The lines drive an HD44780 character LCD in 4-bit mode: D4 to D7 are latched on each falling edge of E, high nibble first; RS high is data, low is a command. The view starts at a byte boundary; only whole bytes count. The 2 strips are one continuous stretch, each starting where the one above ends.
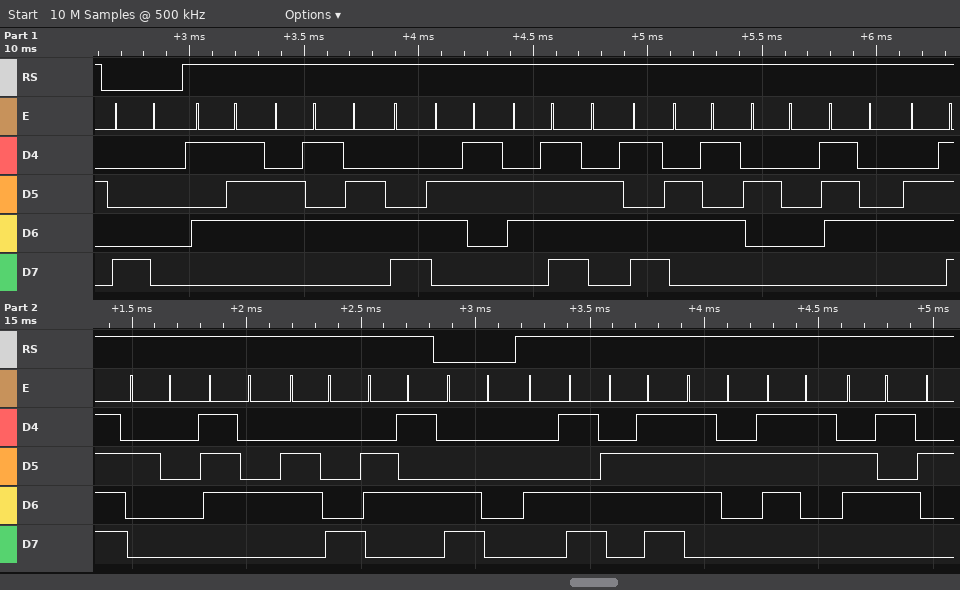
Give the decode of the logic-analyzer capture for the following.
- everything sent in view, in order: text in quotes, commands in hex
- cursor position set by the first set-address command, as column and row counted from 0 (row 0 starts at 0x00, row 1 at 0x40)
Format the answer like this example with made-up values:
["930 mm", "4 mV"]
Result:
["0x80 \"Welcome to the\" 0xC0 \"Morse\"", "column 0, row 0"]
